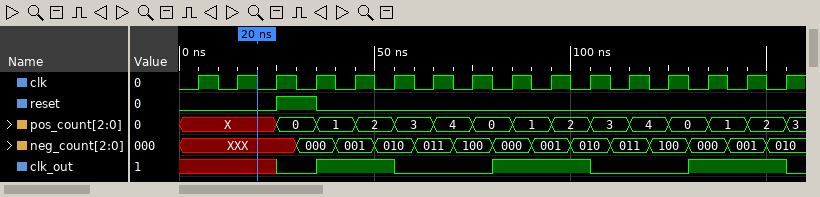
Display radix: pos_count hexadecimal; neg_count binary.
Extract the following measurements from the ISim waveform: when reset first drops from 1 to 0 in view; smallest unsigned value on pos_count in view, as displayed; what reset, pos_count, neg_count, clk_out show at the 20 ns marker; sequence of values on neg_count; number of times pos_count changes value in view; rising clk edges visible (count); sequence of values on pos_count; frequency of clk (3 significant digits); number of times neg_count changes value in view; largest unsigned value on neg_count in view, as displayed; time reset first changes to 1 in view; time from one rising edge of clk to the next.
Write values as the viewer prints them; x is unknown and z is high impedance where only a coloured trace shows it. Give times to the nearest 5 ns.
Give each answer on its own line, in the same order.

35 ns
0
reset=0, pos_count=X, neg_count=XXX, clk_out=x
XXX, 000, 001, 010, 011, 100, 000, 001, 010, 011, 100, 000, 001, 010
14
16
X, 0, 1, 2, 3, 4, 0, 1, 2, 3, 4, 0, 1, 2, 3
100 MHz
13
100
25 ns
10 ns
